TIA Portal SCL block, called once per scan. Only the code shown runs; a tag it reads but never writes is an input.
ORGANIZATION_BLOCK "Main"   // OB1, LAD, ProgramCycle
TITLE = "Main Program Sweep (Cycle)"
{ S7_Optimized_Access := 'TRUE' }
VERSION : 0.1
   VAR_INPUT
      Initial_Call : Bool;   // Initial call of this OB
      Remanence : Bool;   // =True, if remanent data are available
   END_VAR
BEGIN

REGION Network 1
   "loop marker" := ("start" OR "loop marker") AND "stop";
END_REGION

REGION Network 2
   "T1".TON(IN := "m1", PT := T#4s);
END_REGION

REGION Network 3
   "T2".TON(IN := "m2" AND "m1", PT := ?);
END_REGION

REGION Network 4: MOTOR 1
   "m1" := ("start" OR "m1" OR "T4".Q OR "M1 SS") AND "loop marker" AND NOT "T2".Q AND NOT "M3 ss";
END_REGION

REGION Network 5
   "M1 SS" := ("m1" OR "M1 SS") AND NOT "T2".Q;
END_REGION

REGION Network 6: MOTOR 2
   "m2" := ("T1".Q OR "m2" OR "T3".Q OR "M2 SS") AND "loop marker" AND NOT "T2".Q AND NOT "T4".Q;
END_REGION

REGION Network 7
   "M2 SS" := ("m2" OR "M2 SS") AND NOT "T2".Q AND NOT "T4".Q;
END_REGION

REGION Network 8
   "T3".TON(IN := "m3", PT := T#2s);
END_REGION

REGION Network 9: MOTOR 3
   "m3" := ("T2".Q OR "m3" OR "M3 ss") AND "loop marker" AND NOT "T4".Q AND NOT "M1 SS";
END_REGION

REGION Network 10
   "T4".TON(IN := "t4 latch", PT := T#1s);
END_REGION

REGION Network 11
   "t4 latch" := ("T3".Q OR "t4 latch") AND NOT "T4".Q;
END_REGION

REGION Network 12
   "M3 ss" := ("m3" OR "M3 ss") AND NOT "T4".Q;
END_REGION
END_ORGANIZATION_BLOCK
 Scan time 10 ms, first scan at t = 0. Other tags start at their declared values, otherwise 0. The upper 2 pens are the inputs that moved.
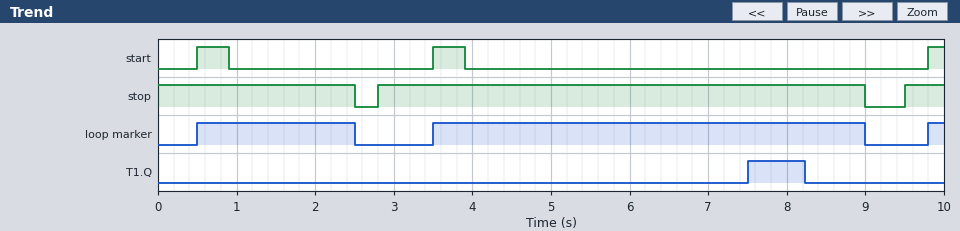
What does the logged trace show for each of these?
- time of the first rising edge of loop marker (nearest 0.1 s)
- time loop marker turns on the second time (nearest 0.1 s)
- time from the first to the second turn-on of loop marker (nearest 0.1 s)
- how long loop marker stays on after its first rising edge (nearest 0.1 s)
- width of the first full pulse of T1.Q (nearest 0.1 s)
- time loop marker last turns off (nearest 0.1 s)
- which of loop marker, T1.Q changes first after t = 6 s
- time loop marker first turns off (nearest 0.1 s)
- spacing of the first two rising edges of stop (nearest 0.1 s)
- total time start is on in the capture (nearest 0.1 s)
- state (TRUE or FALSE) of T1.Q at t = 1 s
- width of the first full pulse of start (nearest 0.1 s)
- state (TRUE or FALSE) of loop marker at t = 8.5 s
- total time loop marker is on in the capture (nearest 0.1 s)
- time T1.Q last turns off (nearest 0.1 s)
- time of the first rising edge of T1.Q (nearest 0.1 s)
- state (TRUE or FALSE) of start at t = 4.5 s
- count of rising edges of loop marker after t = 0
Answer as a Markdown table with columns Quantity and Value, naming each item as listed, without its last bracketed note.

| Quantity | Value |
|---|---|
| time of the first rising edge of loop marker | 0.5 s |
| time loop marker turns on the second time | 3.5 s |
| time from the first to the second turn-on of loop marker | 3.0 s |
| how long loop marker stays on after its first rising edge | 2.0 s |
| width of the first full pulse of T1.Q | 0.7 s |
| time loop marker last turns off | 9.0 s |
| which of loop marker, T1.Q changes first after t = 6 s | T1.Q |
| time loop marker first turns off | 2.5 s |
| spacing of the first two rising edges of stop | 6.7 s |
| total time start is on in the capture | 1.0 s |
| state (TRUE or FALSE) of T1.Q at t = 1 s | FALSE |
| width of the first full pulse of start | 0.4 s |
| state (TRUE or FALSE) of loop marker at t = 8.5 s | TRUE |
| total time loop marker is on in the capture | 7.7 s |
| time T1.Q last turns off | 8.2 s |
| time of the first rising edge of T1.Q | 7.5 s |
| state (TRUE or FALSE) of start at t = 4.5 s | FALSE |
| count of rising edges of loop marker after t = 0 | 3 |
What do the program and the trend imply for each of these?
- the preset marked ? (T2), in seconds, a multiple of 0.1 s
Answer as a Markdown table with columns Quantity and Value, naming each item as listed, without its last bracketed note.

| Quantity | Value |
|---|---|
| the preset marked ? (T2), in seconds, a multiple of 0.1 s | 0.7 s |
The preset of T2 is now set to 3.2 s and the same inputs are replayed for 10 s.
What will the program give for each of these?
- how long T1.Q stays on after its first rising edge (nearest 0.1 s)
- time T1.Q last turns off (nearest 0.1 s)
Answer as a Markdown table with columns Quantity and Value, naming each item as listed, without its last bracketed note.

| Quantity | Value |
|---|---|
| how long T1.Q stays on after its first rising edge | 1.5 s |
| time T1.Q last turns off | 9.0 s |
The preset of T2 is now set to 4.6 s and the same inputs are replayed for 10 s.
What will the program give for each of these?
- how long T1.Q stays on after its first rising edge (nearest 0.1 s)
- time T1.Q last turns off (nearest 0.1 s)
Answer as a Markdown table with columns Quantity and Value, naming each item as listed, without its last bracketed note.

| Quantity | Value |
|---|---|
| how long T1.Q stays on after its first rising edge | 1.5 s |
| time T1.Q last turns off | 9.0 s |
